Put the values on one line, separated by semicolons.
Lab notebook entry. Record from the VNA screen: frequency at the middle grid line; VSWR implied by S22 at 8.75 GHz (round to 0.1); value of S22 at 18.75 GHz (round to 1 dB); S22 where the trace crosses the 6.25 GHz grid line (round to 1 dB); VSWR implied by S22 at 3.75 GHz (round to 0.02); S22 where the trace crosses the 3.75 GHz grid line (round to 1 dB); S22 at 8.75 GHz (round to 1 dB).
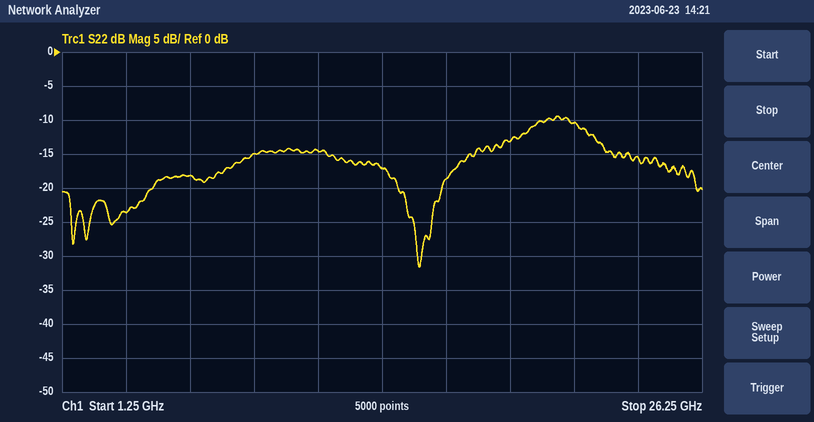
13.75 GHz; 1.4; -13 dB; -18 dB; 1.14; -24 dB; -15 dB
